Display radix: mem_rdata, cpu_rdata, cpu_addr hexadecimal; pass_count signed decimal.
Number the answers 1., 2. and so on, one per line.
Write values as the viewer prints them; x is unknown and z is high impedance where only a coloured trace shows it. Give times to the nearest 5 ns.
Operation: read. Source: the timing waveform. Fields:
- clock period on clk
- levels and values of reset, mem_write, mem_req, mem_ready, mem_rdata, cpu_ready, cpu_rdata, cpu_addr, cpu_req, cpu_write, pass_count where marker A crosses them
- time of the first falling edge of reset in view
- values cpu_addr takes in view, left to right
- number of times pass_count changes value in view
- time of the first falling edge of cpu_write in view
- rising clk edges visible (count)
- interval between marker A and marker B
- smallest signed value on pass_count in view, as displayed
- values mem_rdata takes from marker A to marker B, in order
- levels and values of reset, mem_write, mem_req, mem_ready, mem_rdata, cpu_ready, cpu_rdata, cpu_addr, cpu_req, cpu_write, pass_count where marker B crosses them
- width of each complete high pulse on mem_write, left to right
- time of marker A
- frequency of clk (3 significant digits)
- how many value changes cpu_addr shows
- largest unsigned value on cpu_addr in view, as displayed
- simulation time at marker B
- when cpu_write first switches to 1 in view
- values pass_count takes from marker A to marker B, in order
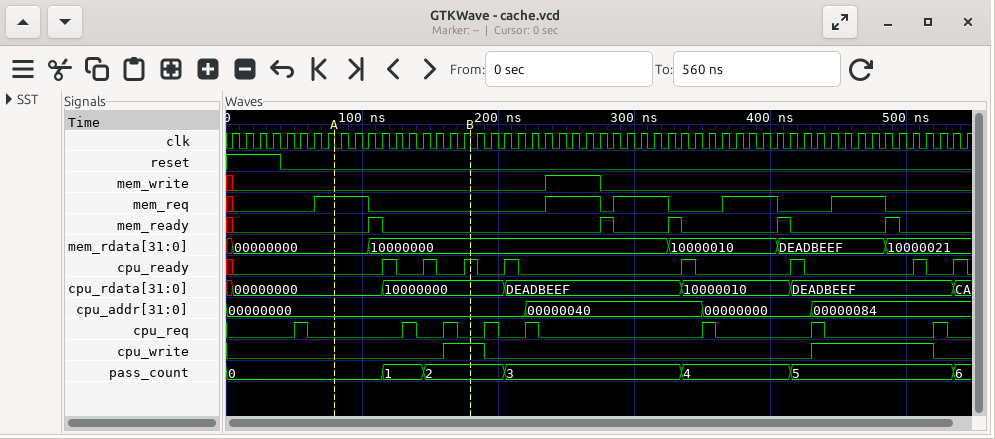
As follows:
1. 10 ns
2. reset=0, mem_write=0, mem_req=1, mem_ready=0, mem_rdata=00000000, cpu_ready=0, cpu_rdata=00000000, cpu_addr=00000000, cpu_req=0, cpu_write=0, pass_count=0
3. 40 ns
4. 00000000, 00000040, 00000000, 00000084
5. 6
6. 190 ns
7. 55
8. 100 ns
9. 0
10. 00000000, 10000000
11. reset=0, mem_write=0, mem_req=0, mem_ready=0, mem_rdata=10000000, cpu_ready=1, cpu_rdata=10000000, cpu_addr=00000000, cpu_req=0, cpu_write=1, pass_count=2
12. 40 ns
13. 80 ns
14. 100 MHz
15. 3
16. 00000084
17. 180 ns
18. 160 ns
19. 0, 1, 2
